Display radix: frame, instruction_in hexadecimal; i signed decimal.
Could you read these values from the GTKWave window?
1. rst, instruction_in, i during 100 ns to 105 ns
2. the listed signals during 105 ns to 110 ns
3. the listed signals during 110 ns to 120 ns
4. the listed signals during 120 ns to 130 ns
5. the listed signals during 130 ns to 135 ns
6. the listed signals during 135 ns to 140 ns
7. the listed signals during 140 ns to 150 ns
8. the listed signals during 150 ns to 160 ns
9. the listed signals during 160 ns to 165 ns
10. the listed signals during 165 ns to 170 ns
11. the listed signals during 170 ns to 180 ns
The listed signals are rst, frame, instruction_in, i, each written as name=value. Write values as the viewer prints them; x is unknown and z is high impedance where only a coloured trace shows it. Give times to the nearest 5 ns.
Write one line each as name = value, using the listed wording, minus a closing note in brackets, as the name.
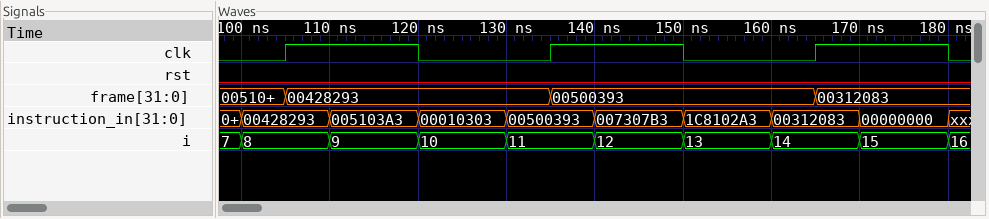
rst, instruction_in, i during 100 ns to 105 ns = rst=0, instruction_in=00428293, i=8
the listed signals during 105 ns to 110 ns = rst=0, frame=00428293, instruction_in=00428293, i=8
the listed signals during 110 ns to 120 ns = rst=0, frame=00428293, instruction_in=005103A3, i=9
the listed signals during 120 ns to 130 ns = rst=0, frame=00428293, instruction_in=00010303, i=10
the listed signals during 130 ns to 135 ns = rst=0, frame=00428293, instruction_in=00500393, i=11
the listed signals during 135 ns to 140 ns = rst=0, frame=00500393, instruction_in=00500393, i=11
the listed signals during 140 ns to 150 ns = rst=0, frame=00500393, instruction_in=007307B3, i=12
the listed signals during 150 ns to 160 ns = rst=0, frame=00500393, instruction_in=1C8102A3, i=13
the listed signals during 160 ns to 165 ns = rst=0, frame=00500393, instruction_in=00312083, i=14
the listed signals during 165 ns to 170 ns = rst=0, frame=00312083, instruction_in=00312083, i=14
the listed signals during 170 ns to 180 ns = rst=0, frame=00312083, instruction_in=00000000, i=15
